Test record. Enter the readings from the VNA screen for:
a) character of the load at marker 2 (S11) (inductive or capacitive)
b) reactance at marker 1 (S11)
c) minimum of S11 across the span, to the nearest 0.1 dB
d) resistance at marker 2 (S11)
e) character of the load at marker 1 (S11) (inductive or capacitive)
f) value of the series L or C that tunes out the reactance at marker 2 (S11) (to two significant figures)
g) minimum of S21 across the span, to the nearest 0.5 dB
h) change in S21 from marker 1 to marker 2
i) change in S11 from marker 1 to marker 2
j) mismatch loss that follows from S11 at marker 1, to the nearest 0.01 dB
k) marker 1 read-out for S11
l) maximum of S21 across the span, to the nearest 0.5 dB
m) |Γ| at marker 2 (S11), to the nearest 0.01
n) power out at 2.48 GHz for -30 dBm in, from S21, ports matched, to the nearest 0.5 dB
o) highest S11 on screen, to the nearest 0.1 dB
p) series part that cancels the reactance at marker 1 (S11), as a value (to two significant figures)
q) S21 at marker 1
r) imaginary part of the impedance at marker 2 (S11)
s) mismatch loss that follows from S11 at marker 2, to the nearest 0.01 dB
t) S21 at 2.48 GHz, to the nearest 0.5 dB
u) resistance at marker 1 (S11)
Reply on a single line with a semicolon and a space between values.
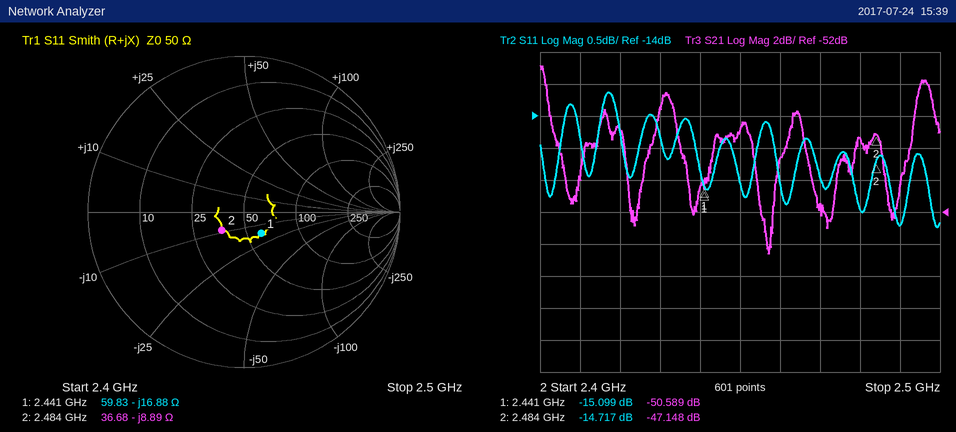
capacitive; -16.88 Ω; -15.7 dB; 36.68 Ω; capacitive; 570 pH; -54.5 dB; 3.441 dB; 0.382 dB; 0.14 dB; -15.099 dB; -43.0 dB; 0.18; -77.5 dBm; -13.6 dB; 1.1 nH; -50.589 dB; -8.89 Ω; 0.15 dB; -47.5 dB; 59.83 Ω
